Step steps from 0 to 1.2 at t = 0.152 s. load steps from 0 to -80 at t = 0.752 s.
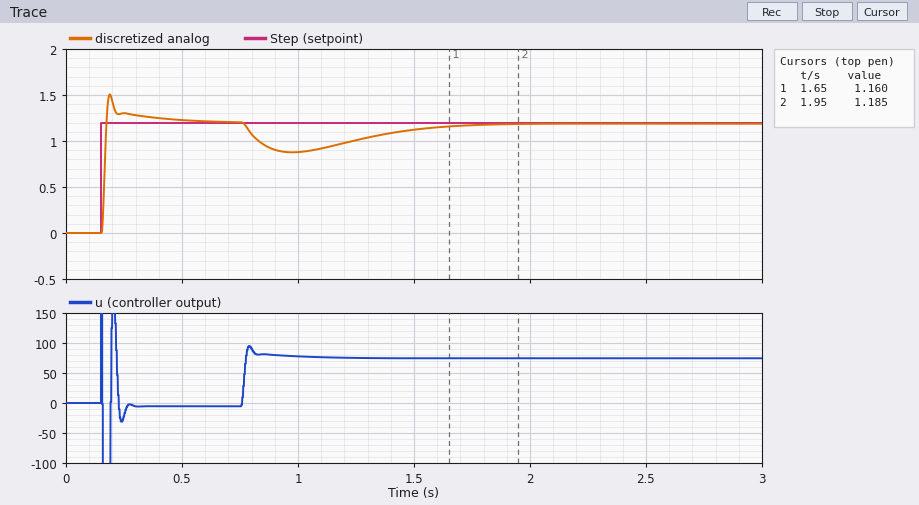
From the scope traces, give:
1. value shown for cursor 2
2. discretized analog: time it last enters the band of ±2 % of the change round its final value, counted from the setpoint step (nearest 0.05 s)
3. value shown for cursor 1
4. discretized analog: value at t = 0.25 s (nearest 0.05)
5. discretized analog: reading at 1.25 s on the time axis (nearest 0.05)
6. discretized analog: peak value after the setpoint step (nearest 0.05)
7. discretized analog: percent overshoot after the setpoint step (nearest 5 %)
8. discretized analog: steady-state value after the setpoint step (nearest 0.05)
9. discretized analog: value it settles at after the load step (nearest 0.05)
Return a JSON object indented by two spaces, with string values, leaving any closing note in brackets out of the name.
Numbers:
{
  "value shown for cursor 2": "1.185",
  "discretized analog: time it last enters the band of ±2 % of the change round its final value, counted from the setpoint step": "0.35 s",
  "value shown for cursor 1": "1.160",
  "discretized analog: value at t = 0.25 s": "1.30",
  "discretized analog: reading at 1.25 s on the time axis": "1.00",
  "discretized analog: peak value after the setpoint step": "1.50",
  "discretized analog: percent overshoot after the setpoint step": "25 %",
  "discretized analog: steady-state value after the setpoint step": "1.20",
  "discretized analog: value it settles at after the load step": "1.20"
}
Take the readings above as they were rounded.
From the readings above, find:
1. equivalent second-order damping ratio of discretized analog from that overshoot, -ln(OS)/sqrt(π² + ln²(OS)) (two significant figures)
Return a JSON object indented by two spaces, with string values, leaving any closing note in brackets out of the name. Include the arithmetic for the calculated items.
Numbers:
{
  "equivalent second-order damping ratio of discretized analog from that overshoot, -ln(OS)/sqrt(π² + ln²(OS))": "ln(0.25) = -1.386; 1.386 / sqrt(9.870 + 1.922) = 0.40"
}
